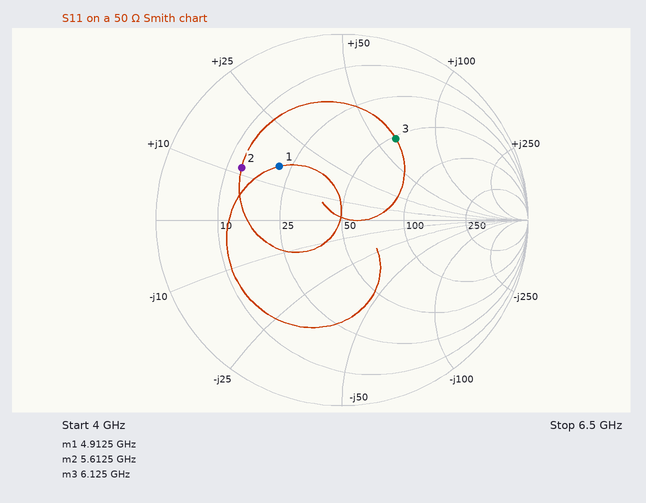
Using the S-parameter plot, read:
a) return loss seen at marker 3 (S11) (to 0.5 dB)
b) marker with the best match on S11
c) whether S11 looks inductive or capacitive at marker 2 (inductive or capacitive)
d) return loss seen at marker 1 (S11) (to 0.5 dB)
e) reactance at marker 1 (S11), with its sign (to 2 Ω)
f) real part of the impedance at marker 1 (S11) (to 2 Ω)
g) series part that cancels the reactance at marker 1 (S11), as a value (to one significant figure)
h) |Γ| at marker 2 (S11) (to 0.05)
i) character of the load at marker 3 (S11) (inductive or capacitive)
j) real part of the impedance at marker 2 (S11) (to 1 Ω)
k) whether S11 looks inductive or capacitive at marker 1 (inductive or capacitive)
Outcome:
5.5 dB
marker 1
inductive
7.0 dB
+16 Ω
22 Ω
2 pF
0.60
inductive
13 Ω
inductive
